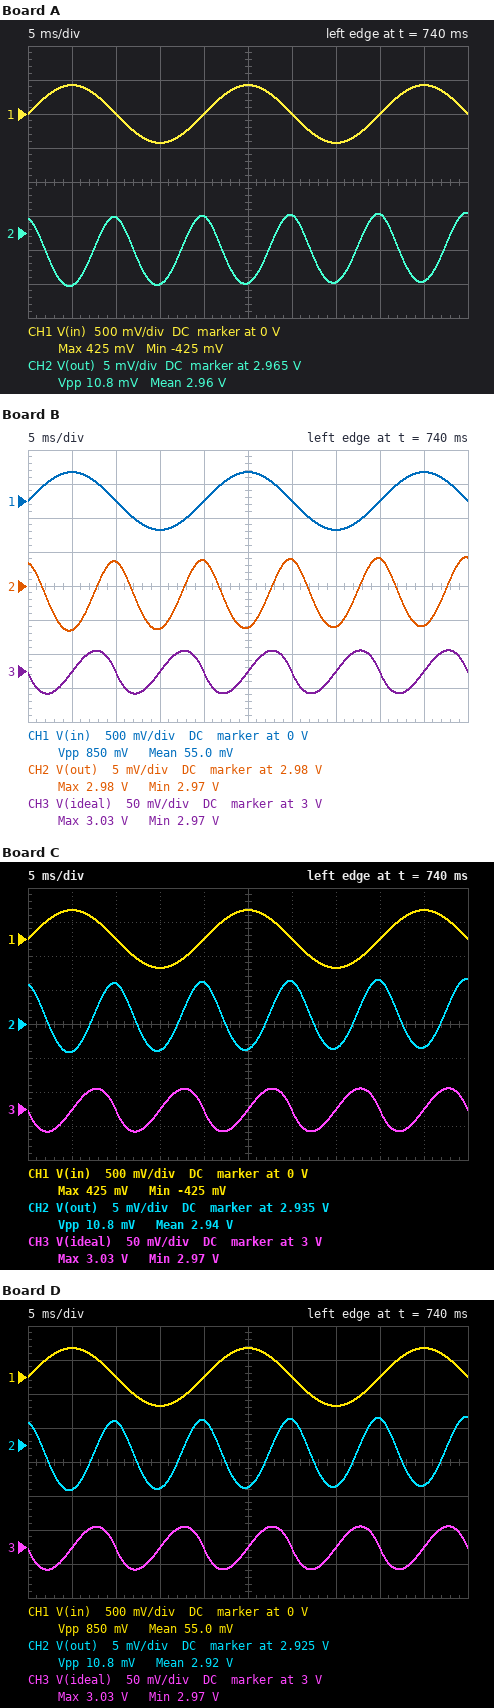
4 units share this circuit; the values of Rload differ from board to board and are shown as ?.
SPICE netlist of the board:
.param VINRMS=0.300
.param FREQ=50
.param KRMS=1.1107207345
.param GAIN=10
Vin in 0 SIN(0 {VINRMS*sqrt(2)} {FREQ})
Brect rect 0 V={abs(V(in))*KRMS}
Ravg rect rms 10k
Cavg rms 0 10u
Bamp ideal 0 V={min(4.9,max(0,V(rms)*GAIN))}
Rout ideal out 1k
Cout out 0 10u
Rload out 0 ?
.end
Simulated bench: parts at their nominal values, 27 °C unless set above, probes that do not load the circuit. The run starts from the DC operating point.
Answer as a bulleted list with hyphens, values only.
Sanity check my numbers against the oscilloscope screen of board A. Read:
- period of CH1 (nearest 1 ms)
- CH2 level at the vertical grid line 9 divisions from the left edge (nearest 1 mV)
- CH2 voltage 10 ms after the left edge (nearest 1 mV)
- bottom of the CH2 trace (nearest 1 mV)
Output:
- 20 ms
- 2.958 V
- 2.967 V
- 2.957 V
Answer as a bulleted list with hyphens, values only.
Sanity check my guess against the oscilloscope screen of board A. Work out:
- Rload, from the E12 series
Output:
- 82 kΩ
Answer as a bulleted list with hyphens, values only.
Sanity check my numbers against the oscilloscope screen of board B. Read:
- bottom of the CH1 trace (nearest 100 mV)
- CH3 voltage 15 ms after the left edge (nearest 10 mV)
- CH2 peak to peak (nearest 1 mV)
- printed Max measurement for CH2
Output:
- -400 mV
- 3.00 V
- 11 mV
- 2.98 V
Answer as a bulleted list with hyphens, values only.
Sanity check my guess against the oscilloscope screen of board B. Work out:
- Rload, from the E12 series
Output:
- 150 kΩ
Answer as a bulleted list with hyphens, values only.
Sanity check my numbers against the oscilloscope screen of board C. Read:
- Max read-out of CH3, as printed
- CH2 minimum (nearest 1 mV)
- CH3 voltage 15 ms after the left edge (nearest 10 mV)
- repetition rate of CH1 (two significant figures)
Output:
- 3.03 V
- 2.931 V
- 3.00 V
- 50 Hz
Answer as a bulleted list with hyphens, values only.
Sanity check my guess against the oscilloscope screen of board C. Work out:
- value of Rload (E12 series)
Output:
- 47 kΩ
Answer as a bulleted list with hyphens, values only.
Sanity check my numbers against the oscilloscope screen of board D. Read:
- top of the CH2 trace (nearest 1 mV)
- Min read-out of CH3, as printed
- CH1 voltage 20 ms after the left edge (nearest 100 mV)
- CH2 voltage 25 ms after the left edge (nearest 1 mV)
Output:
- 2.929 V
- 2.97 V
- 0 V
- 2.919 V
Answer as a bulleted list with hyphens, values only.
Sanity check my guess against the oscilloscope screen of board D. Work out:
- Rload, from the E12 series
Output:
- 39 kΩ
